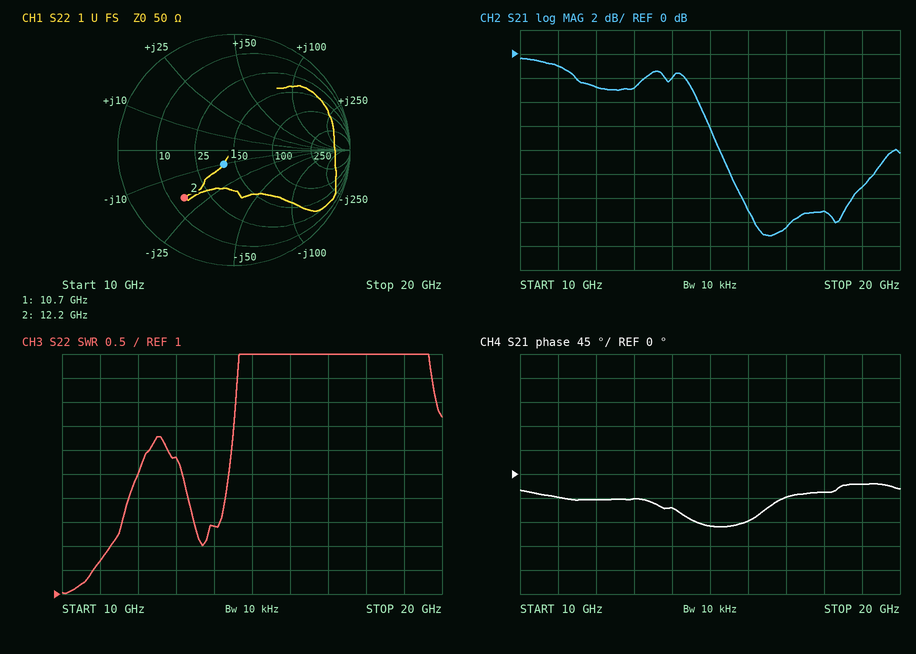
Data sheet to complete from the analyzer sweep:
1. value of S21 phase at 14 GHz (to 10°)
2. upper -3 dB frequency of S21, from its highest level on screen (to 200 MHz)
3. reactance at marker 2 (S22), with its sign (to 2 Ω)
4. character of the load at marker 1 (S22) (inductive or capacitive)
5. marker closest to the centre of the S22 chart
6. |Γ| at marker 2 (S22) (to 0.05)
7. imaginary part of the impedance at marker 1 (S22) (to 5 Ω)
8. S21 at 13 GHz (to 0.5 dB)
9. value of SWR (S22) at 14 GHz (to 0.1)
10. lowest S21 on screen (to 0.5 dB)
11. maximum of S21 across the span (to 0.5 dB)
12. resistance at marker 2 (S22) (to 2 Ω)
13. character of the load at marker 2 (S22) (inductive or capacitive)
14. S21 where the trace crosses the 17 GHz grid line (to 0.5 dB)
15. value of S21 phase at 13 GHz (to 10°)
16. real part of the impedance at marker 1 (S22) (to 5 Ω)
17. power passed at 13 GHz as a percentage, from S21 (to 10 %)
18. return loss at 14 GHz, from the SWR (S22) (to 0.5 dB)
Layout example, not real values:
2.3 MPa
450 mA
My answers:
-60°
14.6 GHz
-18 Ω
capacitive
marker 1
0.60
-10 Ω
-3.0 dB
2.4
-15.0 dB
-0.5 dB
14 Ω
capacitive
-14.5 dB
-50°
40 Ω
50 %
7.5 dB
